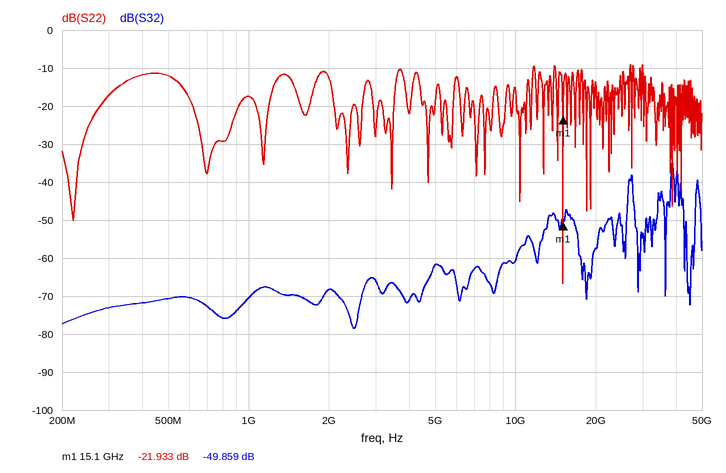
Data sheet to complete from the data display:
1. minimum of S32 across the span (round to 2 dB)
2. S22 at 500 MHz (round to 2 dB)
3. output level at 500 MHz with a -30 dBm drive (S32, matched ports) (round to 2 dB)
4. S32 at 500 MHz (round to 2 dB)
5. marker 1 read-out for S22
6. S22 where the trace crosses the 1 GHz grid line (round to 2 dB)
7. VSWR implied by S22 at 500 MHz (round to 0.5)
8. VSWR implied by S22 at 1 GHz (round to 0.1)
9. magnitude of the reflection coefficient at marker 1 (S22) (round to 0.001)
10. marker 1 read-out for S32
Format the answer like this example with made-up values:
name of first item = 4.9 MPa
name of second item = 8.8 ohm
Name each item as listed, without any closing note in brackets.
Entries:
minimum of S32 across the span = -78 dB
S22 at 500 MHz = -12 dB
output level at 500 MHz with a -30 dBm drive (S32, matched ports) = -100 dBm
S32 at 500 MHz = -70 dB
marker 1 read-out for S22 = -21.933 dB
S22 where the trace crosses the 1 GHz grid line = -18 dB
VSWR implied by S22 at 500 MHz = 1.5
VSWR implied by S22 at 1 GHz = 1.3
magnitude of the reflection coefficient at marker 1 (S22) = 0.080
marker 1 read-out for S32 = -49.859 dB
